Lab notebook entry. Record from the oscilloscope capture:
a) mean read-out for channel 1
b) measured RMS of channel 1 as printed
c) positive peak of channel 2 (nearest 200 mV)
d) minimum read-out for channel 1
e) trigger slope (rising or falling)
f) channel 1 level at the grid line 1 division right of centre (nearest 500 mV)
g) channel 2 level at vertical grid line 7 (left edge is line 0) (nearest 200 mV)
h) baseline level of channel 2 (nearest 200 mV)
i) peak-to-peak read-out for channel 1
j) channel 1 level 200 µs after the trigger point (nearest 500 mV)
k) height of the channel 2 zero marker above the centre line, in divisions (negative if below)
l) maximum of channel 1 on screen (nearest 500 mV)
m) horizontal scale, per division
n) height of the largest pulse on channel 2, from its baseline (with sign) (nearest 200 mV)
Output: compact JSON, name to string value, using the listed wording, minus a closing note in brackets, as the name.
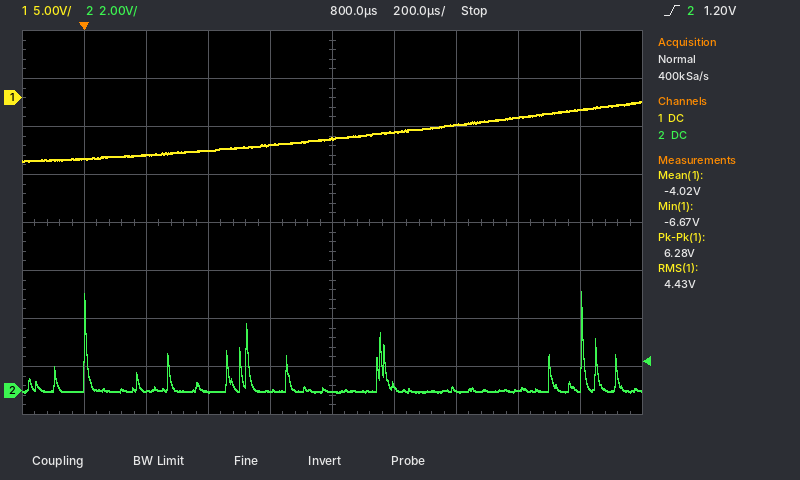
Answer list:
{"mean read-out for channel 1": "-4.02 V", "measured RMS of channel 1 as printed": "4.43 V", "positive peak of channel 2": "4.2 V", "minimum read-out for channel 1": "-6.67 V", "trigger slope": "rising", "channel 1 level at the grid line 1 division right of centre": "-3.5 V", "channel 2 level at vertical grid line 7 (left edge is line 0)": "0.0 V", "baseline level of channel 2": "0.0 V", "peak-to-peak read-out for channel 1": "6.28 V", "channel 1 level 200 µs after the trigger point": "-6.0 V", "height of the channel 2 zero marker above the centre line, in divisions": "-3.5 div", "maximum of channel 1 on screen": "-500 mV", "horizontal scale, per division": "200 µs", "height of the largest pulse on channel 2, from its baseline (with sign)": "+4.2 V"}
